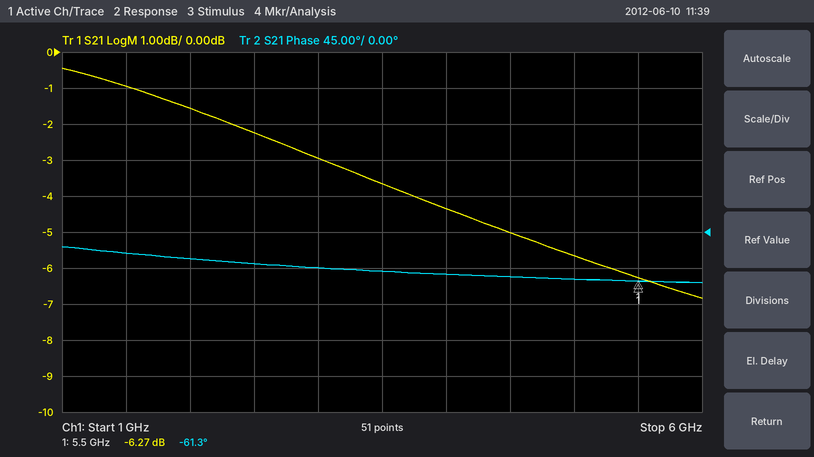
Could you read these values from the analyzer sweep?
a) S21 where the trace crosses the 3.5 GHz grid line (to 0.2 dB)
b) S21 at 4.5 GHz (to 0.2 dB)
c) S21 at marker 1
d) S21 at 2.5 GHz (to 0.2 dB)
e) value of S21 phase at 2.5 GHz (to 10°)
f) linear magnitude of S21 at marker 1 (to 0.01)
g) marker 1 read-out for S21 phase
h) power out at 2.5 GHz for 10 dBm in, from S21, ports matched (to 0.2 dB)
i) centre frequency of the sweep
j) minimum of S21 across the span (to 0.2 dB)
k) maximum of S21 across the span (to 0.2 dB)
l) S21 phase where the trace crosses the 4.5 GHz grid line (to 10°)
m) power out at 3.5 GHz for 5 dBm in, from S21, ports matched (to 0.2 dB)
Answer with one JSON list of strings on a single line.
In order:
["-3.6 dB", "-5.0 dB", "-6.27 dB", "-2.2 dB", "-40°", "0.49", "-61.3°", "7.8 dBm", "3.5 GHz", "-6.8 dB", "-0.4 dB", "-60°", "1.4 dBm"]
